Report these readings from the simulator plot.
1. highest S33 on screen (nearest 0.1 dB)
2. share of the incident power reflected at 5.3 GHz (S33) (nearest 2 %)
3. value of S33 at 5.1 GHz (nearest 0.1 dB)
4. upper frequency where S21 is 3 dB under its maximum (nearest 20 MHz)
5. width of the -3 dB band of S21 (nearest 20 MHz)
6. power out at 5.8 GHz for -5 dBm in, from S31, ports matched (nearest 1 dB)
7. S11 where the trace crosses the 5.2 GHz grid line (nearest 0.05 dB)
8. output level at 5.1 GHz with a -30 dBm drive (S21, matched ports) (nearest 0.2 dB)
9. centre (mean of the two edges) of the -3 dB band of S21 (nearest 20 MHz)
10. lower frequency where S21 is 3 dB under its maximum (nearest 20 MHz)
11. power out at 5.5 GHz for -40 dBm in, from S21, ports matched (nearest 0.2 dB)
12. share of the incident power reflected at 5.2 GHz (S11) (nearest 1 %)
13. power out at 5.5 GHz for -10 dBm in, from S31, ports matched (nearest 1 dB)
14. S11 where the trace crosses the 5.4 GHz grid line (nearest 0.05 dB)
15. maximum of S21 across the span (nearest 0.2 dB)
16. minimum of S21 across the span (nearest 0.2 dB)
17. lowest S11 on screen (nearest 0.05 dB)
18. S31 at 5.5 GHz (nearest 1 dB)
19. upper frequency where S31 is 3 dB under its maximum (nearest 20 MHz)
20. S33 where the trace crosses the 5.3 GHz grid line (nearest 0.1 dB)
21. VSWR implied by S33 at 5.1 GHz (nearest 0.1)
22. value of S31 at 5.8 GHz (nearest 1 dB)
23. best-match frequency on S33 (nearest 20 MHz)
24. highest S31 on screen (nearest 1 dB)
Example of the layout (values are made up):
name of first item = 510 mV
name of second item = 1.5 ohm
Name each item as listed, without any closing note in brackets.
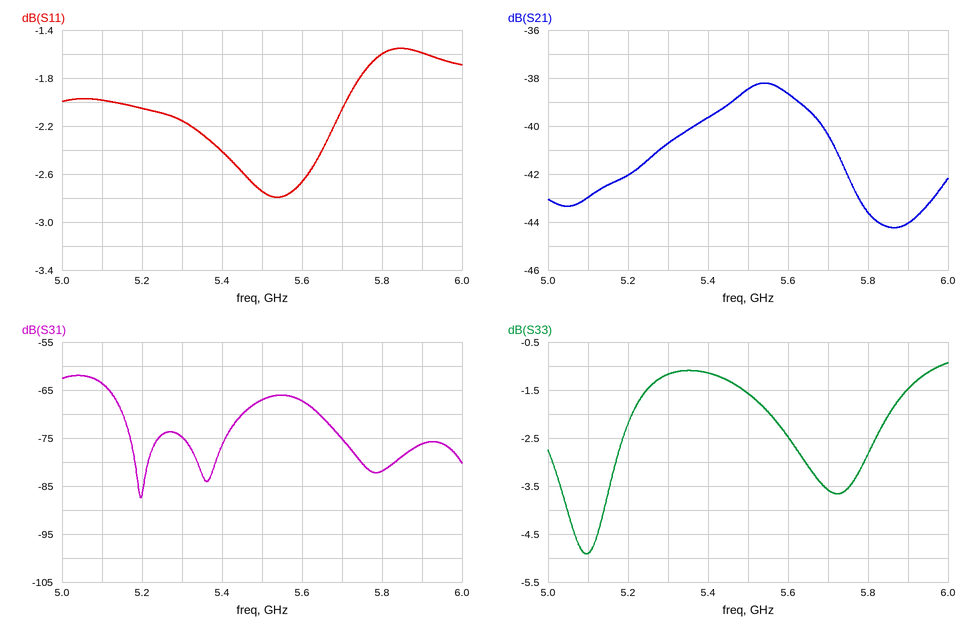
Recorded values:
highest S33 on screen = -0.9 dB
share of the incident power reflected at 5.3 GHz (S33) = 76 %
value of S33 at 5.1 GHz = -4.9 dB
upper frequency where S21 is 3 dB under its maximum = 5.72 GHz
width of the -3 dB band of S21 = 460 MHz
power out at 5.8 GHz for -5 dBm in, from S31, ports matched = -87 dBm
S11 where the trace crosses the 5.2 GHz grid line = -2.05 dB
output level at 5.1 GHz with a -30 dBm drive (S21, matched ports) = -73.0 dBm
centre (mean of the two edges) of the -3 dB band of S21 = 5.50 GHz
lower frequency where S21 is 3 dB under its maximum = 5.26 GHz
power out at 5.5 GHz for -40 dBm in, from S21, ports matched = -78.4 dBm
share of the incident power reflected at 5.2 GHz (S11) = 62 %
power out at 5.5 GHz for -10 dBm in, from S31, ports matched = -77 dBm
S11 where the trace crosses the 5.4 GHz grid line = -2.40 dB
maximum of S21 across the span = -38.2 dB
minimum of S21 across the span = -44.2 dB
lowest S11 on screen = -2.80 dB
S31 at 5.5 GHz = -67 dB
upper frequency where S31 is 3 dB under its maximum = 5.12 GHz
S33 where the trace crosses the 5.3 GHz grid line = -1.2 dB
VSWR implied by S33 at 5.1 GHz = 3.6
value of S31 at 5.8 GHz = -82 dB
best-match frequency on S33 = 5.10 GHz
highest S31 on screen = -62 dB
